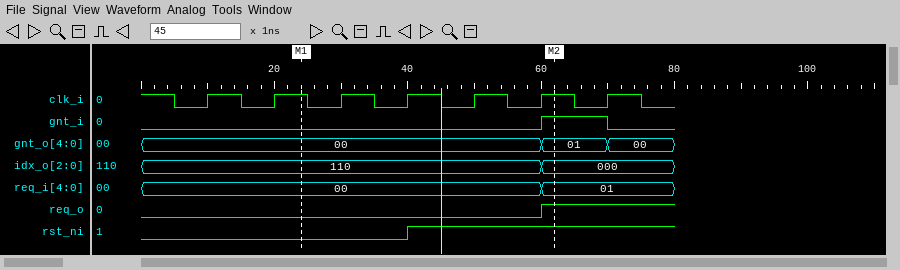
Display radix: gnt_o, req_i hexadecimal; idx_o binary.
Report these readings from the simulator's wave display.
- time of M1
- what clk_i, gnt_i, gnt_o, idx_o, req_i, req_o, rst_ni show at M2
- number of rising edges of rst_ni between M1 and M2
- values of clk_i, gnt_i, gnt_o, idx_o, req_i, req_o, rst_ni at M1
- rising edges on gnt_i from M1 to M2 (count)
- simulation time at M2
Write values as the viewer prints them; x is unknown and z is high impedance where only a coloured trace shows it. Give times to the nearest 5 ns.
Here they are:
25 ns
clk_i=1, gnt_i=1, gnt_o=01, idx_o=000, req_i=01, req_o=1, rst_ni=1
1
clk_i=1, gnt_i=0, gnt_o=00, idx_o=110, req_i=00, req_o=0, rst_ni=0
1
60 ns
